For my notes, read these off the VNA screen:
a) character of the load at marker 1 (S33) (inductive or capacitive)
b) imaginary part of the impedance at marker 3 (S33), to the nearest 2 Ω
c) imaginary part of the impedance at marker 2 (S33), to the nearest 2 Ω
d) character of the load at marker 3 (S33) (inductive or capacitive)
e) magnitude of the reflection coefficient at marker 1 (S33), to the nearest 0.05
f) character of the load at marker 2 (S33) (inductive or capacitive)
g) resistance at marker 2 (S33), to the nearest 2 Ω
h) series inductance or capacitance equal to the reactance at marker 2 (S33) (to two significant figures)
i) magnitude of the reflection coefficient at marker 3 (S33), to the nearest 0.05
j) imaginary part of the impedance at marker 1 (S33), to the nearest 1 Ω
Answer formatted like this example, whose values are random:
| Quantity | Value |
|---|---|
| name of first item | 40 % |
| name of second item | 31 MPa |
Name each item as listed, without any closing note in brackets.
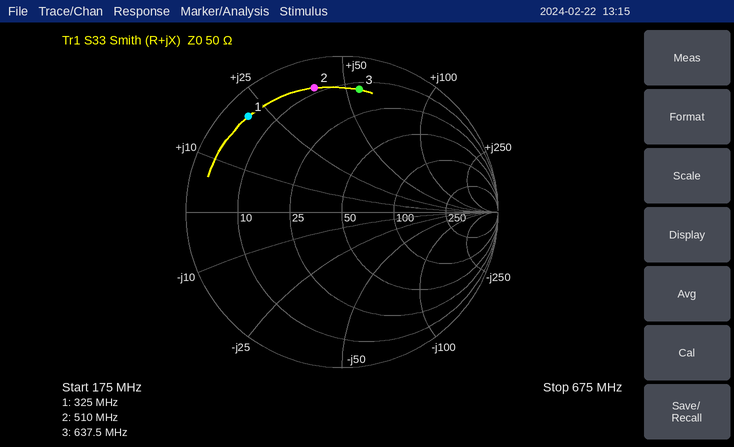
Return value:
| Quantity | Value |
|---|---|
| character of the load at marker 1 (S33) | inductive |
| imaginary part of the impedance at marker 3 (S33), to the nearest 2 Ω | +56 Ω |
| imaginary part of the impedance at marker 2 (S33), to the nearest 2 Ω | +40 Ω |
| character of the load at marker 3 (S33) | inductive |
| magnitude of the reflection coefficient at marker 1 (S33), to the nearest 0.05 | 0.85 |
| character of the load at marker 2 (S33) | inductive |
| resistance at marker 2 (S33), to the nearest 2 Ω | 8 Ω |
| series inductance or capacitance equal to the reactance at marker 2 (S33) | 12 nH |
| magnitude of the reflection coefficient at marker 3 (S33), to the nearest 0.05 | 0.80 |
| imaginary part of the impedance at marker 1 (S33), to the nearest 1 Ω | +21 Ω |
